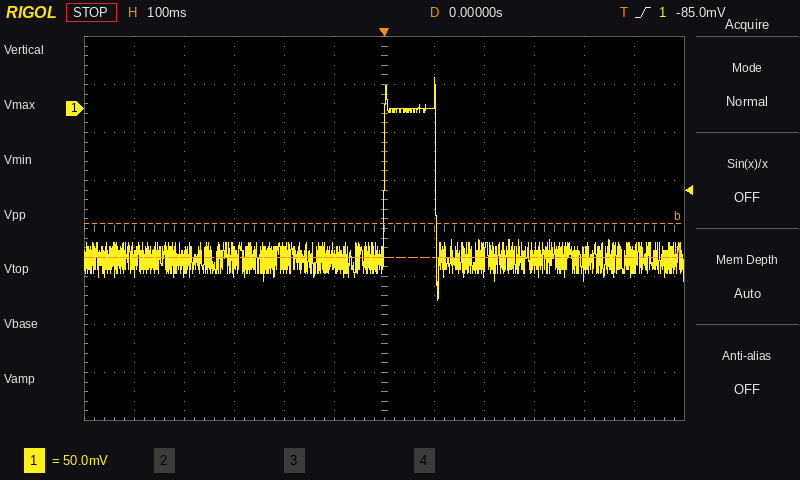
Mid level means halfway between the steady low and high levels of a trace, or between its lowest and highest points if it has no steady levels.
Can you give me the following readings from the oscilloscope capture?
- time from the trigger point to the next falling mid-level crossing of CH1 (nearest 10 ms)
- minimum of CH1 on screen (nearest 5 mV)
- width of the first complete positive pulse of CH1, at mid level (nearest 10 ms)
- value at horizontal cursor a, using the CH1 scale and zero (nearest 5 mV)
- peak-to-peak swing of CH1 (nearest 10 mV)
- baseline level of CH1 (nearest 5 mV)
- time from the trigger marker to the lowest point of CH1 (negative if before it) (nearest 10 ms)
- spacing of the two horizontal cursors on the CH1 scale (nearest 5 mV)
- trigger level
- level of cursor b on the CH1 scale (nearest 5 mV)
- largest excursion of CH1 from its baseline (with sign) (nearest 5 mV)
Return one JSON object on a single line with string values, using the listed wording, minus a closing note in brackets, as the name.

{"time from the trigger point to the next falling mid-level crossing of CH1": "100 ms", "minimum of CH1 on screen": "-200 mV", "width of the first complete positive pulse of CH1, at mid level": "100 ms", "value at horizontal cursor a, using the CH1 scale and zero": "-155 mV", "peak-to-peak swing of CH1": "230 mV", "baseline level of CH1": "-155 mV", "time from the trigger marker to the lowest point of CH1 (negative if before it)": "+110 ms", "spacing of the two horizontal cursors on the CH1 scale": "35 mV", "trigger level": "-85.0 mV", "level of cursor b on the CH1 scale": "-120 mV", "largest excursion of CH1 from its baseline (with sign)": "+190 mV"}
